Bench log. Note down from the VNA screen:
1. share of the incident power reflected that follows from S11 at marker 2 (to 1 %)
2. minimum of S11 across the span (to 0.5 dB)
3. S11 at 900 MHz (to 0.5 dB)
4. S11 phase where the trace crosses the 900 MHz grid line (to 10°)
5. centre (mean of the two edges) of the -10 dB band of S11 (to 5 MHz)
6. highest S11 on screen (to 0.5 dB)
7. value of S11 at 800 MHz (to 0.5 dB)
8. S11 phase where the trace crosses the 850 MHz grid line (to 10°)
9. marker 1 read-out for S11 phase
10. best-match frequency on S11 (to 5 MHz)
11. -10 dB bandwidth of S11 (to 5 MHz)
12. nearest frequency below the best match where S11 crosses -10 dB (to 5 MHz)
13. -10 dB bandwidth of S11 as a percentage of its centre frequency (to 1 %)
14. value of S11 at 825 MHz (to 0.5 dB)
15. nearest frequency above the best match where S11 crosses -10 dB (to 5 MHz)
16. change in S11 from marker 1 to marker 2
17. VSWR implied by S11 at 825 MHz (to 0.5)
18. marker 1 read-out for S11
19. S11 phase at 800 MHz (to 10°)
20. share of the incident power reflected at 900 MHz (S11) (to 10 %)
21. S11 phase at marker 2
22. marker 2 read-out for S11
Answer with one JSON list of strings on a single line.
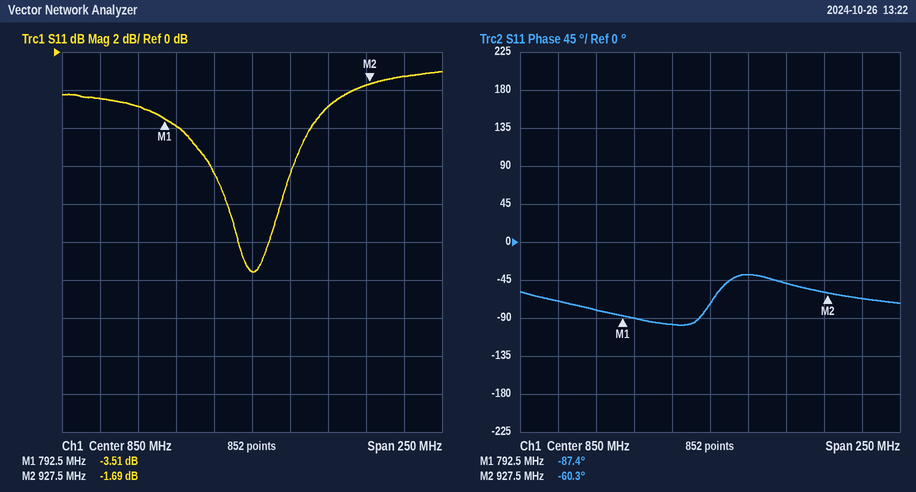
["68 %", "-11.5 dB", "-3.0 dB", "-50°", "850 MHz", "-1.0 dB", "-4.0 dB", "-70°", "-87.4°", "850 MHz", "20 MHz", "840 MHz", "2 %", "-6.5 dB", "860 MHz", "1.82 dB", "3.0", "-3.51 dB", "-90°", "50 %", "-60.3°", "-1.69 dB"]
